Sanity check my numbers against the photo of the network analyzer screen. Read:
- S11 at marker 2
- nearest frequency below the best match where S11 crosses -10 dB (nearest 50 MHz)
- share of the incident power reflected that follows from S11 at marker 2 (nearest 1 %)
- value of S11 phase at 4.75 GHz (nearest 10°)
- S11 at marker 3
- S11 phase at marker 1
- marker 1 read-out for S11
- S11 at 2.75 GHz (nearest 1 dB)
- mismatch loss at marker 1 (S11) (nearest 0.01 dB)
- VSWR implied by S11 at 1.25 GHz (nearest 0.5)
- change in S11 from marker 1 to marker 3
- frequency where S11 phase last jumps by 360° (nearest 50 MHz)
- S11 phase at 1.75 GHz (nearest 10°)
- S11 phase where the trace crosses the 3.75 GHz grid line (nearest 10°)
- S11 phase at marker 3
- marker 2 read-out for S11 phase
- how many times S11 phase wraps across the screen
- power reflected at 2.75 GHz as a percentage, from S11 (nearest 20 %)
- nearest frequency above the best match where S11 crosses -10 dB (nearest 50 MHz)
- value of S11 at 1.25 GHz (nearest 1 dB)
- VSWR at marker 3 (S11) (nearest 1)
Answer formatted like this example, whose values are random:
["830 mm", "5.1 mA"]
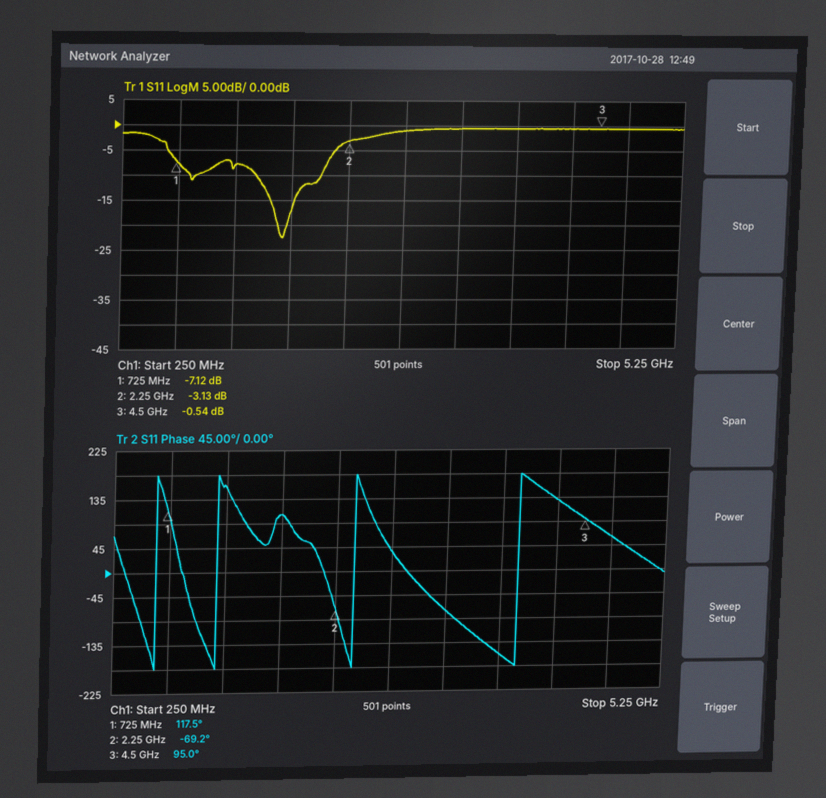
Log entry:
["-3.13 dB", "1.45 GHz", "49 %", "60°", "-0.54 dB", "117.5°", "-7.12 dB", "-1 dB", "0.94 dB", "2.5", "6.58 dB", "3.90 GHz", "110°", "-160°", "95.0°", "-69.2°", "4", "80 %", "2.00 GHz", "-8 dB", "32"]
